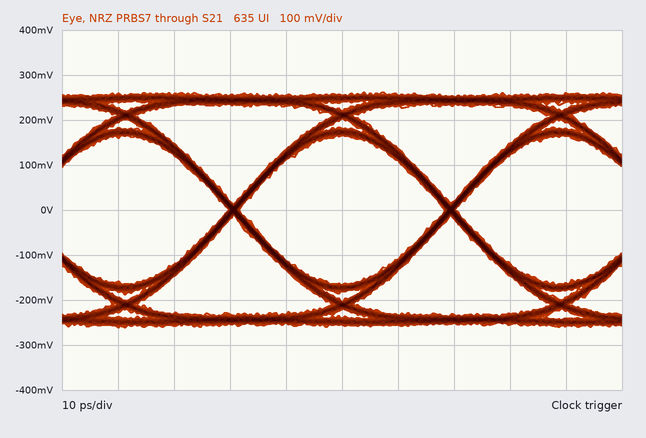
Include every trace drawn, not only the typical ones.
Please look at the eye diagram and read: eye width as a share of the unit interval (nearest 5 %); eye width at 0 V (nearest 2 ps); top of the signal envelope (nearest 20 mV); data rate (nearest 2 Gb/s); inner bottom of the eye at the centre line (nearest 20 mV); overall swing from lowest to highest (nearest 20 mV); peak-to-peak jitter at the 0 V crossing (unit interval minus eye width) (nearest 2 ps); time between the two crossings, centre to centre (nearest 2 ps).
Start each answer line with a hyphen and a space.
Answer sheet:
- 95 %
- 36 ps
- 260 mV
- 26 Gb/s
- -160 mV
- 520 mV
- 2 ps
- 38 ps
